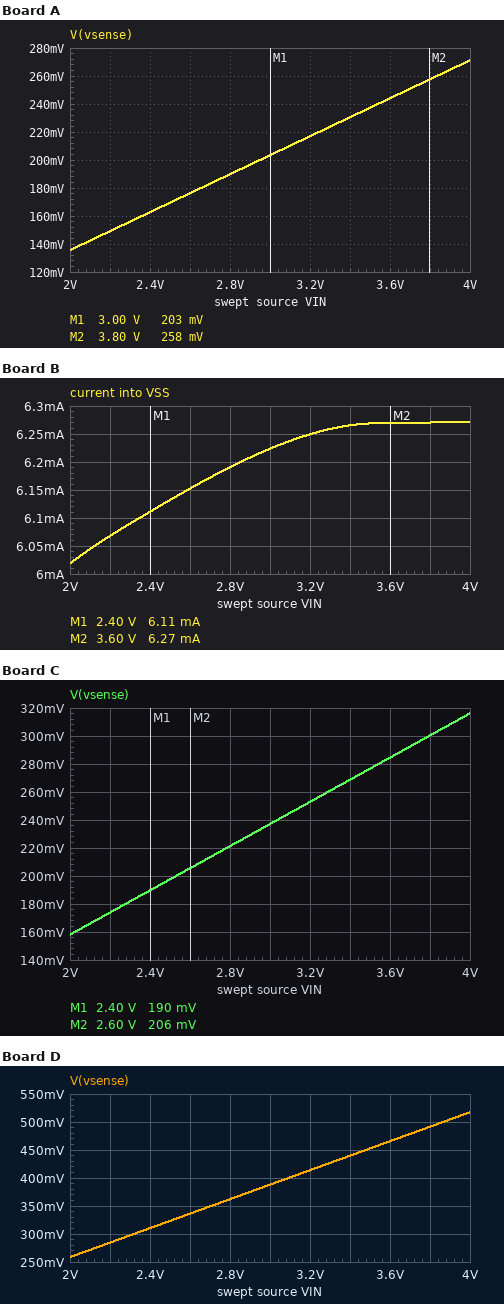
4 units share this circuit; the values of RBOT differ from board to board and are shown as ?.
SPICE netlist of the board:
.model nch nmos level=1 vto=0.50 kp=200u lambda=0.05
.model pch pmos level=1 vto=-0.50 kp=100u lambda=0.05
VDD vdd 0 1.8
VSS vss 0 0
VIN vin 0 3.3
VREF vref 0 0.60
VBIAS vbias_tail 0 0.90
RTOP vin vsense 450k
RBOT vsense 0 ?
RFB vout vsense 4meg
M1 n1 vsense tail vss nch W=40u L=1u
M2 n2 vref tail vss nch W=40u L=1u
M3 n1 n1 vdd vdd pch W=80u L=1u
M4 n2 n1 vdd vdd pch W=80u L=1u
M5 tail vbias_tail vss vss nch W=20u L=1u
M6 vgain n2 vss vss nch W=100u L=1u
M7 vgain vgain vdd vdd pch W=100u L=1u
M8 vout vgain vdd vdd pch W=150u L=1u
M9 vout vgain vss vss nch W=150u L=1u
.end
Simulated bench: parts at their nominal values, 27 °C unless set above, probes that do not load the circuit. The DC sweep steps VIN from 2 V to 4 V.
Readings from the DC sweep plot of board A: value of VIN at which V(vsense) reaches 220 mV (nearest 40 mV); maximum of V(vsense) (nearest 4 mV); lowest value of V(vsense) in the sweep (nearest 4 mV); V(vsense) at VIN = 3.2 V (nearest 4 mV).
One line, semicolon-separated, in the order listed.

3.24 V; 272 mV; 136 mV; 216 mV
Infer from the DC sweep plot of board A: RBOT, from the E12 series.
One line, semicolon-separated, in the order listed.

33 kΩ
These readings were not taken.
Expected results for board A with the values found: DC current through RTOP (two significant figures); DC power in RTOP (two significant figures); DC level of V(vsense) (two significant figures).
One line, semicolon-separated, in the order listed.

6.8 µA; 21 µW; 220 mV
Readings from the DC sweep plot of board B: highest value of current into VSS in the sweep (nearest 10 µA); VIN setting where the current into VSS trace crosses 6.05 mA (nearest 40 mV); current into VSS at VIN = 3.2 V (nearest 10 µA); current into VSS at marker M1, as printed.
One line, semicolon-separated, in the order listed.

6.27 mA; 2.12 V; 6.25 mA; 6.11 mA
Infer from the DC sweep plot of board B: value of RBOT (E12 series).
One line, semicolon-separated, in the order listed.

220 kΩ
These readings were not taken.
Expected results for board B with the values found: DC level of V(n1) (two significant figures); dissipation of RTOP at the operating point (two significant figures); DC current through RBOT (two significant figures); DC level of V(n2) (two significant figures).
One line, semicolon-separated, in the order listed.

1.0 V; 11 µW; 5.0 µA; 1.8 V
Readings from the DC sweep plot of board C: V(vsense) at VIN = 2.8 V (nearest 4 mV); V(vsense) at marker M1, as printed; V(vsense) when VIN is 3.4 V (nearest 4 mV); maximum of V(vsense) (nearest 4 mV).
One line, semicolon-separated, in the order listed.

220 mV; 190 mV; 268 mV; 316 mV
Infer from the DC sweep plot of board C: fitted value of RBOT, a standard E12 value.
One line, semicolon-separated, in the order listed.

39 kΩ
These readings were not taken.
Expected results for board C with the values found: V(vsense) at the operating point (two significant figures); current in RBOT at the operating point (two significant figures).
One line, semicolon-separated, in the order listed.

260 mV; 6.7 µA
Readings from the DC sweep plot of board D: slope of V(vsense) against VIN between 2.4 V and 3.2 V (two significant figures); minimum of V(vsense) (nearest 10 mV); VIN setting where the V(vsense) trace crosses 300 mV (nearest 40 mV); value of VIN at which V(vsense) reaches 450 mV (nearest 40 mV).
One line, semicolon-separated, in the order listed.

0.13 V/V; 260 mV; 2.32 V; 3.48 V
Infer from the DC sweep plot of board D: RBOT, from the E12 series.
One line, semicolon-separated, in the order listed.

68 kΩ
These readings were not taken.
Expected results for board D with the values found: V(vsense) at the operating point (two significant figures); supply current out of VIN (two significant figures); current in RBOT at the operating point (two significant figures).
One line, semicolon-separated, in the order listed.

430 mV; 6.4 µA; 6.3 µA
